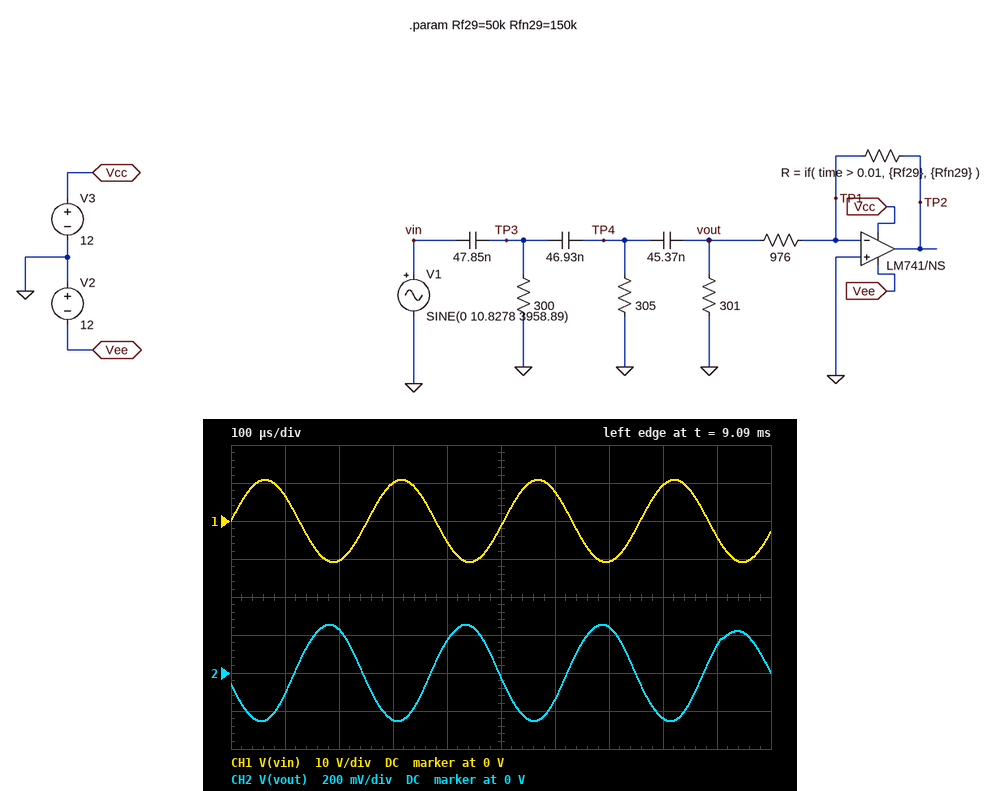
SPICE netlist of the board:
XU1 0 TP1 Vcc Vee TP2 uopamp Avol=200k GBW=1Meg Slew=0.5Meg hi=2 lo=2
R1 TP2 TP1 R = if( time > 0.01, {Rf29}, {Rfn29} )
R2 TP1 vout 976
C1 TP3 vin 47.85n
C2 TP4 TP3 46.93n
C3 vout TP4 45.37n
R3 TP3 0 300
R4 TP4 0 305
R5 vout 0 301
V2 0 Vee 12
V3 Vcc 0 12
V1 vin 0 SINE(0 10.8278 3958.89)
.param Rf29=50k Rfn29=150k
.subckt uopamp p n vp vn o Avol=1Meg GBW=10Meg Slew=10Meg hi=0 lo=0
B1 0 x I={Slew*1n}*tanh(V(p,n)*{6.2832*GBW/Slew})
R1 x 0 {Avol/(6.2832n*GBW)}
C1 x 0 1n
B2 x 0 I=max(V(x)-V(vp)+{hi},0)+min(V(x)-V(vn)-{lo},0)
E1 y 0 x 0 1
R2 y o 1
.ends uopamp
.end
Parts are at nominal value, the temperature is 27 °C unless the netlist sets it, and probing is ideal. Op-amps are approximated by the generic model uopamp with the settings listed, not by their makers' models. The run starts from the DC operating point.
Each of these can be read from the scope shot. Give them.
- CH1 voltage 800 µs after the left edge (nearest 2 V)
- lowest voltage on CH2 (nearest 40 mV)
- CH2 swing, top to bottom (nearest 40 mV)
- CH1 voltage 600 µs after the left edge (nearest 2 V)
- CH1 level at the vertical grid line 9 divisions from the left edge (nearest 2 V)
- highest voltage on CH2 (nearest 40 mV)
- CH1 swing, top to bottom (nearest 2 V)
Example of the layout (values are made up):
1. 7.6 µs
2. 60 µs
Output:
1. 10 V
2. -240 mV
3. 520 mV
4. 8 V
5. -4 V
6. 240 mV
7. 22 V
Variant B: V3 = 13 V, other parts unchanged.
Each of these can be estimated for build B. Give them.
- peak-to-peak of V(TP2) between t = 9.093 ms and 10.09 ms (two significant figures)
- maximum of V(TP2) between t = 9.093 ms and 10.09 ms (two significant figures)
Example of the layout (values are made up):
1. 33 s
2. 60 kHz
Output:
1. 21 V
2. 11 V
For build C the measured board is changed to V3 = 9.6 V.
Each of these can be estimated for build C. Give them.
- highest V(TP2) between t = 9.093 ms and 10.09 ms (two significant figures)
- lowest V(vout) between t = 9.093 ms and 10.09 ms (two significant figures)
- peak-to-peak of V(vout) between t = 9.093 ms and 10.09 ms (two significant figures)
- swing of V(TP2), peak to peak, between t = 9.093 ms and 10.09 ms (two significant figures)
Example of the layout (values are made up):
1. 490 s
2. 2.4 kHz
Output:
1. 7.6 V
2. -260 mV
3. 510 mV
4. 18 V
